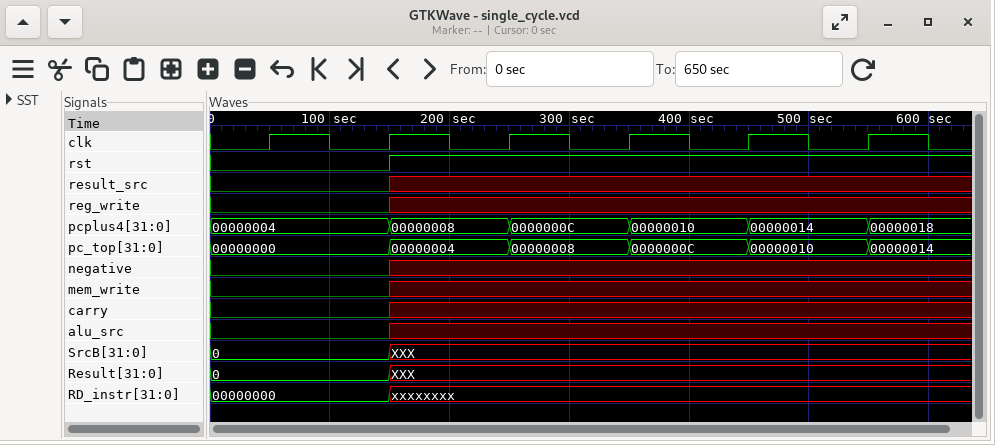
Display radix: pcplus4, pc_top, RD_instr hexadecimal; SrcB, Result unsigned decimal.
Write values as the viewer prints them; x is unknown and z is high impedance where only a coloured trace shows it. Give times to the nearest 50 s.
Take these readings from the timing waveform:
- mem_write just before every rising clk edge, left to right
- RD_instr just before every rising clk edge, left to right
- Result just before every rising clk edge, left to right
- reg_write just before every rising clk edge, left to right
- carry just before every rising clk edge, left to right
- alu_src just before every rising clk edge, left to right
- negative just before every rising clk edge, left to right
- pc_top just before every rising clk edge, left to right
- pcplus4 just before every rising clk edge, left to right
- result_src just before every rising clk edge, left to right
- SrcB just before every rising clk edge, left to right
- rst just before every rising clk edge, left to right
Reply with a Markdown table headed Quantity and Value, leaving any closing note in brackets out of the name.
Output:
| Quantity | Value |
|---|---|
| mem_write just before every rising clk edge, left to right | 0 0 x x x x |
| RD_instr just before every rising clk edge, left to right | 00000000, 00000000, xxxxxxxx, xxxxxxxx, xxxxxxxx, xxxxxxxx |
| Result just before every rising clk edge, left to right | 0, 0, XXX, XXX, XXX, XXX |
| reg_write just before every rising clk edge, left to right | 0 0 x x x x |
| carry just before every rising clk edge, left to right | 0 0 x x x x |
| alu_src just before every rising clk edge, left to right | 0 0 x x x x |
| negative just before every rising clk edge, left to right | 0 0 x x x x |
| pc_top just before every rising clk edge, left to right | 00000000, 00000000, 00000004, 00000008, 0000000C, 00000010 |
| pcplus4 just before every rising clk edge, left to right | 00000004, 00000004, 00000008, 0000000C, 00000010, 00000014 |
| result_src just before every rising clk edge, left to right | 0 0 x x x x |
| SrcB just before every rising clk edge, left to right | 0, 0, XXX, XXX, XXX, XXX |
| rst just before every rising clk edge, left to right | 0 0 1 1 1 1 |
